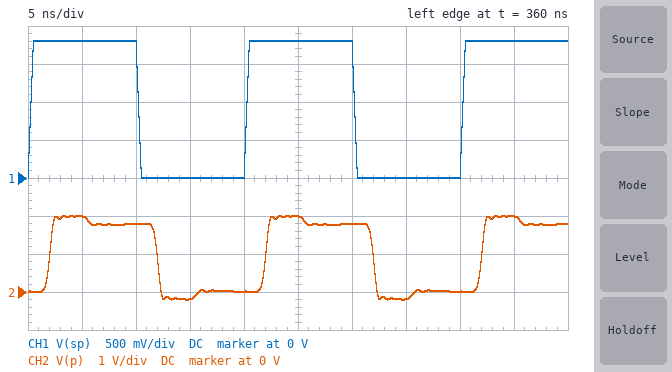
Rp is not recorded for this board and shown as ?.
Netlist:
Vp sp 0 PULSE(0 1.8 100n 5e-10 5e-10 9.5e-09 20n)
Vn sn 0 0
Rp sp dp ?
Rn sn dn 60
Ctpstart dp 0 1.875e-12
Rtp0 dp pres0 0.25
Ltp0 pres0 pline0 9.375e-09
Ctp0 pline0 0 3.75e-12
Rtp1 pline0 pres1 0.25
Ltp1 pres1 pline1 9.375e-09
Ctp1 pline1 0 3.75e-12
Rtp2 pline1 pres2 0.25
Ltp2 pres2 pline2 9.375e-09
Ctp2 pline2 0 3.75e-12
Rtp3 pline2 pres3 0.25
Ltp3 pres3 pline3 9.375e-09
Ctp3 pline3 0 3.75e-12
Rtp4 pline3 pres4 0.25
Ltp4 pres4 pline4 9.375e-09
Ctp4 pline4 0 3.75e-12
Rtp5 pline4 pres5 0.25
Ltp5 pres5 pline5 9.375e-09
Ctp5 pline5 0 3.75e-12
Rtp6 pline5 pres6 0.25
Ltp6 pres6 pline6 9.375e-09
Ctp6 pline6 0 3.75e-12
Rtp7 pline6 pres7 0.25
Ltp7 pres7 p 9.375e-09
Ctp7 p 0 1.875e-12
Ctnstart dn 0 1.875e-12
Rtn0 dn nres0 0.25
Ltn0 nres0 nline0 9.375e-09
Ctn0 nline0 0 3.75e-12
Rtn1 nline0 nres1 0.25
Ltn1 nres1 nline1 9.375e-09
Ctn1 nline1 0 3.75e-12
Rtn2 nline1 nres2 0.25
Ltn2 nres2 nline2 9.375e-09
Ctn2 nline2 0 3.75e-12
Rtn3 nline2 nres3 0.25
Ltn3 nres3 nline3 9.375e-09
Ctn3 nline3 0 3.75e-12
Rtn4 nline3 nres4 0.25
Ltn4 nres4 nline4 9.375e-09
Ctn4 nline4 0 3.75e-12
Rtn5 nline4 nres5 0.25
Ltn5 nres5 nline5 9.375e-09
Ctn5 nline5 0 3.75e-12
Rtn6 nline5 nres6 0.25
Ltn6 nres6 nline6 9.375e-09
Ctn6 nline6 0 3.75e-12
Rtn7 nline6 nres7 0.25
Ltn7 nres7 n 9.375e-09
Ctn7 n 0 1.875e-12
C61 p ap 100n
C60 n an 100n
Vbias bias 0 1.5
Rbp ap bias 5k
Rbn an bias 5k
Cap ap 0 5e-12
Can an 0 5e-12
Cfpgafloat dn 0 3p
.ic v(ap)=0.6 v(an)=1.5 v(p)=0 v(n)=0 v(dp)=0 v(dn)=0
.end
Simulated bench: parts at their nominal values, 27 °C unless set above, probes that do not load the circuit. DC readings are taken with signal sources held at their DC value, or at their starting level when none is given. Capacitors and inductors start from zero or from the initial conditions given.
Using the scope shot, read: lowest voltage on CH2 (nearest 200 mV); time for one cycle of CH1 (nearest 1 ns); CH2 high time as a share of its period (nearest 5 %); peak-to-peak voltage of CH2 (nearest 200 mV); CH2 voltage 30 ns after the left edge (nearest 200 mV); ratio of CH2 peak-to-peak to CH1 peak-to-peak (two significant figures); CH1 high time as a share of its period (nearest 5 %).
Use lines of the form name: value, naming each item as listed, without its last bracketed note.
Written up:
lowest voltage on CH2: -200 mV
time for one cycle of CH1: 20 ns
CH2 high time as a share of its period: 50 %
peak-to-peak voltage of CH2: 2.2 V
CH2 voltage 30 ns after the left edge: 1.8 V
ratio of CH2 peak-to-peak to CH1 peak-to-peak: 1.2
CH1 high time as a share of its period: 50 %
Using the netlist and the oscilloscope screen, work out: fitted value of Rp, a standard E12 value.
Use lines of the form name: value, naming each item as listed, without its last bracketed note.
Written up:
fitted value of Rp, a standard E12 value: 39 Ω
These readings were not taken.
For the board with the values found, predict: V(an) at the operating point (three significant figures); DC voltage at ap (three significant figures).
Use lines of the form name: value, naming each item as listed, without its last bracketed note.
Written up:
V(an) at the operating point: 1.50 V
DC voltage at ap: 1.50 V
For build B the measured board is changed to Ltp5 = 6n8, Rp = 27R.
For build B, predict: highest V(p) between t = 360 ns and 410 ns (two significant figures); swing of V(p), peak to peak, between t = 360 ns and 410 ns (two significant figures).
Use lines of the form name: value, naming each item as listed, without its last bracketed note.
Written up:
highest V(p) between t = 360 ns and 410 ns: 2.3 V
swing of V(p), peak to peak, between t = 360 ns and 410 ns: 2.9 V
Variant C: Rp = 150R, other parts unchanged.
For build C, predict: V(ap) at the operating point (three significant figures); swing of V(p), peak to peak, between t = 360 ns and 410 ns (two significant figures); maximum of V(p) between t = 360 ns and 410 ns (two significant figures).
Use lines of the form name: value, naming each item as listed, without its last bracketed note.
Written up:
V(ap) at the operating point: 1.50 V
swing of V(p), peak to peak, between t = 360 ns and 410 ns: 1.4 V
maximum of V(p) between t = 360 ns and 410 ns: 1.6 V
